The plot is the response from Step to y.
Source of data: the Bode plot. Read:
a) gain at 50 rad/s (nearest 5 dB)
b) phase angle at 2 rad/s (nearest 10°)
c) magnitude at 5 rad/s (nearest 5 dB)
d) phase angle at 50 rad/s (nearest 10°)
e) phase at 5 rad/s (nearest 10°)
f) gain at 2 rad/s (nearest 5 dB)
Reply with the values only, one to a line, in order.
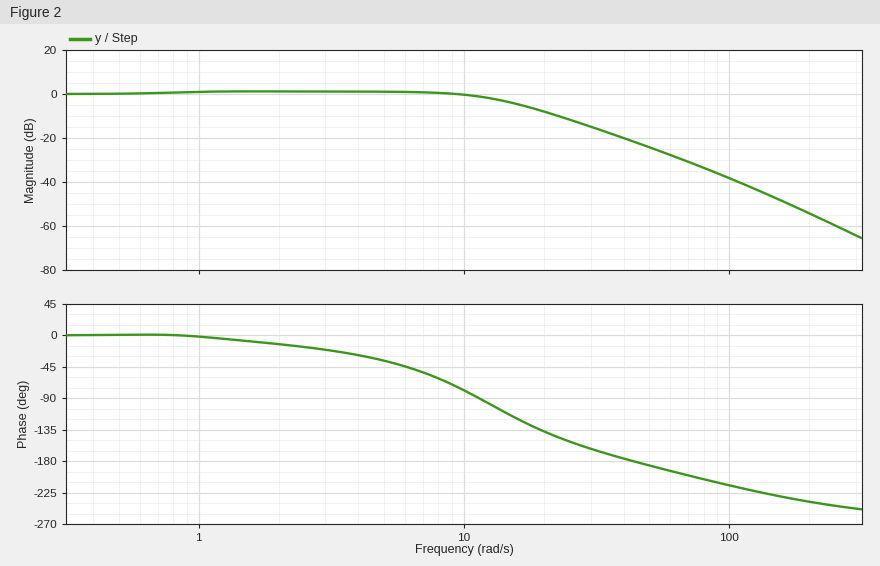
-25 dB
-10°
0 dB
-190°
-40°
0 dB
